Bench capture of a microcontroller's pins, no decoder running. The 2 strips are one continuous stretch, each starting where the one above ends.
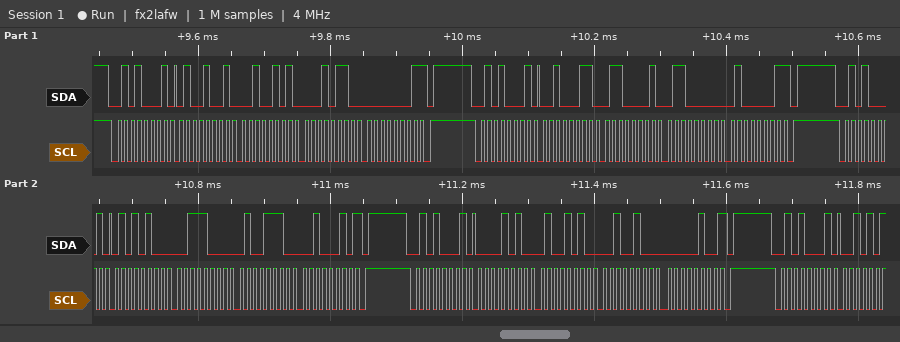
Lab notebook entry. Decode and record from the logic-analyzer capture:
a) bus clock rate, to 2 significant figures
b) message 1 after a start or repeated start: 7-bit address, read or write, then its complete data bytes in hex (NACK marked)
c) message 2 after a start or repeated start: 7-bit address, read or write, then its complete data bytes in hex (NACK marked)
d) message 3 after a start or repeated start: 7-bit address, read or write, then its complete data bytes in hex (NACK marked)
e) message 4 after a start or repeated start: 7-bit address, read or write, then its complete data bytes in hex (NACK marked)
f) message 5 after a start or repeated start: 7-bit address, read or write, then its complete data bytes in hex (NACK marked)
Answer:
100 kHz
0x28 read: 49 25 16 01 NACK
0x28 read: 23 61 60 41 NACK
0x28 read: 54 38 4E 22 NACK
0x28 read: 0A 4A 24 04 NACK
0x28 read
